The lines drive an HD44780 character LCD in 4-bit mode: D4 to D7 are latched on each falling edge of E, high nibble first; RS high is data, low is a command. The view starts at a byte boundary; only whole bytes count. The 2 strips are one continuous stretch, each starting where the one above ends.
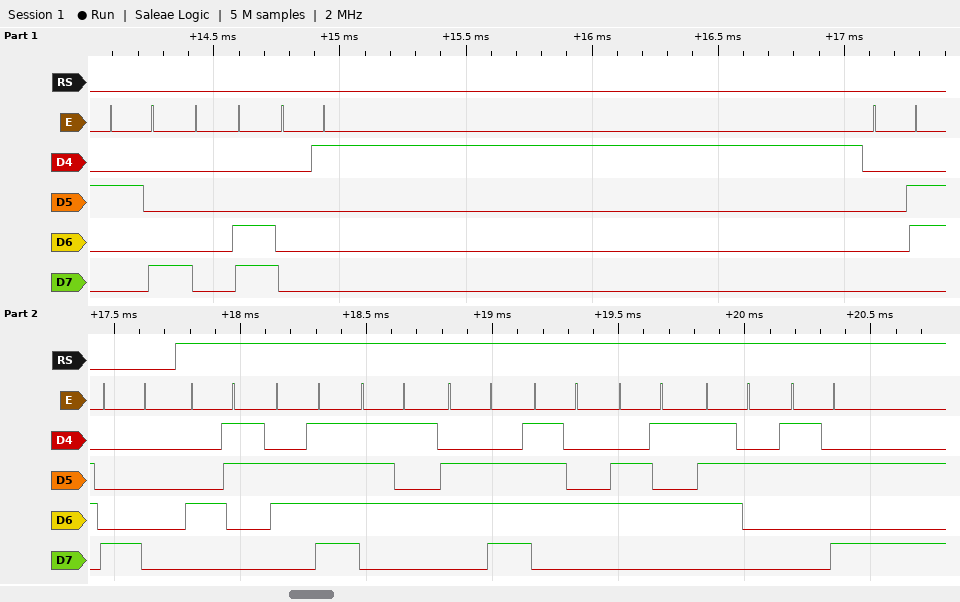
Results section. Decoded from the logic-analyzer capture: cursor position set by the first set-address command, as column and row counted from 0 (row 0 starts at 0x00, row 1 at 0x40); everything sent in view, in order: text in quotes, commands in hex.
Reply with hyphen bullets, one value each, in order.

- column 0, row 0
- 0x28 0x0C 0x01 0x06 0x80 "Counter:"
